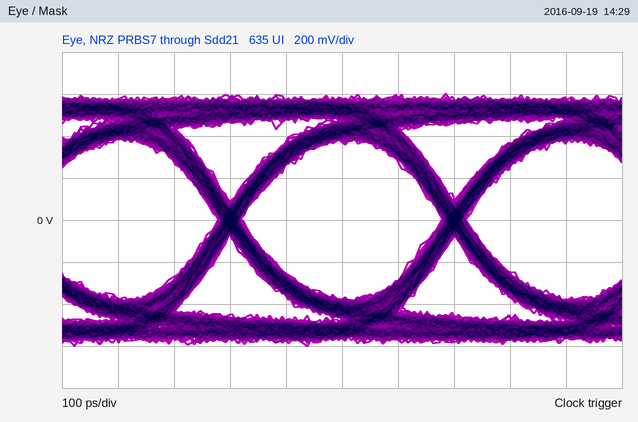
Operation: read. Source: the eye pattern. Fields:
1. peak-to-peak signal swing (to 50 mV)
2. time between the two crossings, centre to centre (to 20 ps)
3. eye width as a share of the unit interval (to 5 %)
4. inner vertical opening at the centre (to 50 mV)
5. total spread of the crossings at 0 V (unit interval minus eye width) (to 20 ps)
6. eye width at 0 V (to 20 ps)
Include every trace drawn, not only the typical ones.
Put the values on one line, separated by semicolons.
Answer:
1.20 V; 400 ps; 90 %; 750 mV; 40 ps; 360 ps
